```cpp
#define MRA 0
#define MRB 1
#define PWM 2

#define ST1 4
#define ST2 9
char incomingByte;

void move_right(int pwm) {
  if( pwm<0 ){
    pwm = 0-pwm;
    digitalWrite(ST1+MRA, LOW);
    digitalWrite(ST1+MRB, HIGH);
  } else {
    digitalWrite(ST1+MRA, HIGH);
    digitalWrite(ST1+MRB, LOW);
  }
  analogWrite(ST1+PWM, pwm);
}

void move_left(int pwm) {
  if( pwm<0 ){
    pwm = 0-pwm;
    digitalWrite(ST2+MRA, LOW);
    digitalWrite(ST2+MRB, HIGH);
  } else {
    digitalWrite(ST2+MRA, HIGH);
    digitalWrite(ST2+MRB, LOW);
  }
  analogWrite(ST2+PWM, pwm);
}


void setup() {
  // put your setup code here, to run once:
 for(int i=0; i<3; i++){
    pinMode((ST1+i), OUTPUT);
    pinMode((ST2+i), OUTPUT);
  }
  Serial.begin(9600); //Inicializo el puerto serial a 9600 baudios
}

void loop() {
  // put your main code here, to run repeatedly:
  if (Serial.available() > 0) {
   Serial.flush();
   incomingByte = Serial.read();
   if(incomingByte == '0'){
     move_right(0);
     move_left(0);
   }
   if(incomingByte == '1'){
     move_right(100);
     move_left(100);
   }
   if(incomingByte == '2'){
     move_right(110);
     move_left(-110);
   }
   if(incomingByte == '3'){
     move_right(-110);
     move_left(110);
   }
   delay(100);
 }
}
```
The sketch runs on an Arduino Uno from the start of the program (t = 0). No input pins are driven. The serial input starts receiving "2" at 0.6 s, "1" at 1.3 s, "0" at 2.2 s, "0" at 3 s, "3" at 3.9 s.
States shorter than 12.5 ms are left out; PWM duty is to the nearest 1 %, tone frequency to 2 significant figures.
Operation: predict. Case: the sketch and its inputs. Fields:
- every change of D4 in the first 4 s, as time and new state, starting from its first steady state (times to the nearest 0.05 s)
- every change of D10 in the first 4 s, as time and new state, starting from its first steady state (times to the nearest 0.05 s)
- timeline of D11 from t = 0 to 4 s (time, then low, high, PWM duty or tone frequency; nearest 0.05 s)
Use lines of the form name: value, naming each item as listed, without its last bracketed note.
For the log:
every change of D4 in the first 4 s, as time and new state, starting from its first steady state: 0 s low; 0.6 s high; 3.9 s low
every change of D10 in the first 4 s, as time and new state, starting from its first steady state: 0 s low; 0.6 s high; 1.3 s low
timeline of D11 from t = 0 to 4 s: 0 s low; 0.6 s PWM 43 %; 1.3 s PWM 39 %; 2.2 s low; 3.9 s PWM 43 %
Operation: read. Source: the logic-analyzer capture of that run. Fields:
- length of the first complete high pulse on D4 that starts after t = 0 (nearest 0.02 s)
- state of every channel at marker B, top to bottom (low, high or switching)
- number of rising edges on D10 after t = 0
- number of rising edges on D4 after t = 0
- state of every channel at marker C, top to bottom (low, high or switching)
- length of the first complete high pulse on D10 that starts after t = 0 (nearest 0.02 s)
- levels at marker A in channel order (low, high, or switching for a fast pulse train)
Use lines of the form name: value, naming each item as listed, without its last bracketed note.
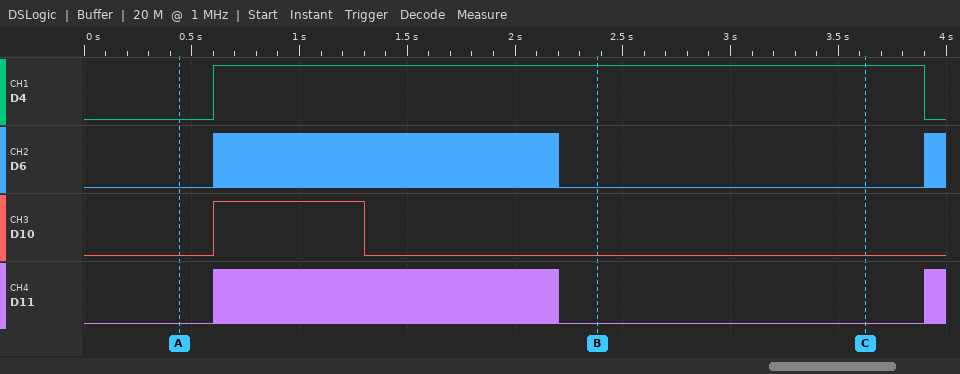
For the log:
length of the first complete high pulse on D4 that starts after t = 0: 3.30 s
state of every channel at marker B, top to bottom: D4 high, D6 low, D10 low, D11 low
number of rising edges on D10 after t = 0: 1
number of rising edges on D4 after t = 0: 1
state of every channel at marker C, top to bottom: D4 high, D6 low, D10 low, D11 low
length of the first complete high pulse on D10 that starts after t = 0: 0.70 s
levels at marker A in channel order: D4 low, D6 low, D10 low, D11 low
